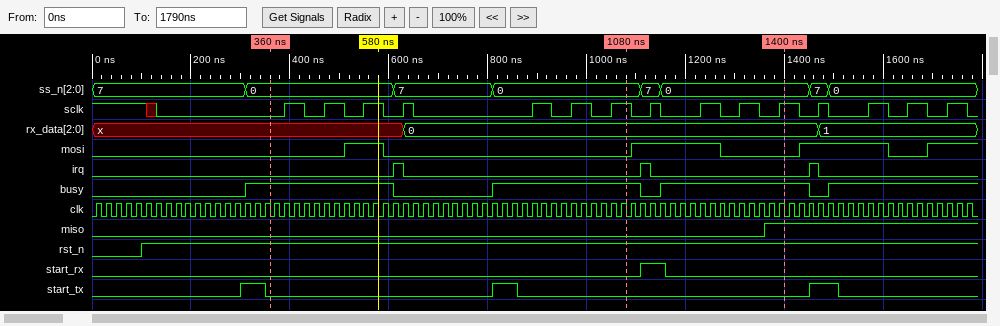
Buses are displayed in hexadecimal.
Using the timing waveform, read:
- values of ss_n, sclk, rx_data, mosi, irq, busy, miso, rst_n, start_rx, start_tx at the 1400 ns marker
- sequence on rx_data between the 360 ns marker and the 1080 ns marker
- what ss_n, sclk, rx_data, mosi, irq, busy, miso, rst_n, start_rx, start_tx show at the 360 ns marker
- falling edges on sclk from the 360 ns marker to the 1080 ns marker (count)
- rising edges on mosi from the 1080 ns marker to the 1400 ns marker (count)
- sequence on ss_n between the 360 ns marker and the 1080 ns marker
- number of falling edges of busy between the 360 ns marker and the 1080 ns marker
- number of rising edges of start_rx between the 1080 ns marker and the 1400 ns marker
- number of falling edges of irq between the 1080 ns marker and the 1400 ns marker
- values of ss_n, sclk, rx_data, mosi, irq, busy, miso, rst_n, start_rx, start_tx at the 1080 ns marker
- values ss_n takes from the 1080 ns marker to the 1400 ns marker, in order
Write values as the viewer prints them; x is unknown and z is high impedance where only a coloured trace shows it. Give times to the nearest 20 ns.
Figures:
ss_n=0, sclk=1, rx_data=0, mosi=0, irq=0, busy=1, miso=1, rst_n=1, start_rx=0, start_tx=0
x, 0
ss_n=0, sclk=0, rx_data=x, mosi=0, irq=0, busy=1, miso=0, rst_n=1, start_rx=0, start_tx=0
6
1
0, 7, 0
1
1
1
ss_n=0, sclk=1, rx_data=0, mosi=0, irq=0, busy=1, miso=0, rst_n=1, start_rx=0, start_tx=0
0, 7, 0
